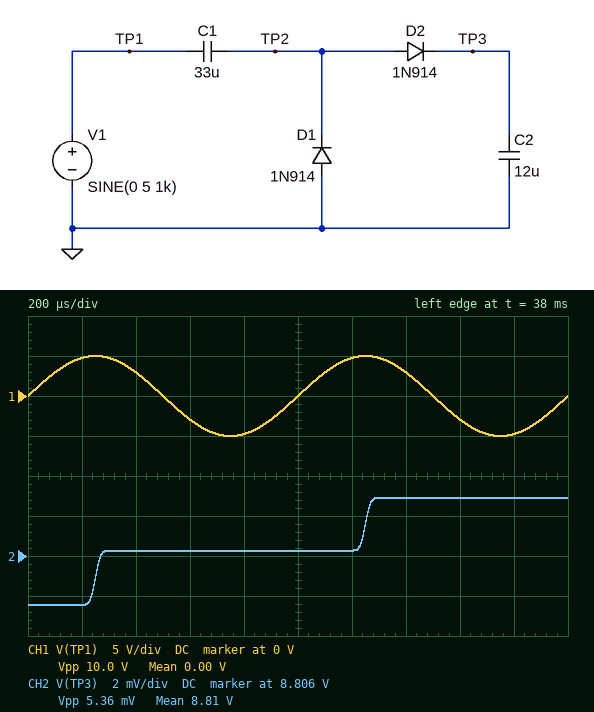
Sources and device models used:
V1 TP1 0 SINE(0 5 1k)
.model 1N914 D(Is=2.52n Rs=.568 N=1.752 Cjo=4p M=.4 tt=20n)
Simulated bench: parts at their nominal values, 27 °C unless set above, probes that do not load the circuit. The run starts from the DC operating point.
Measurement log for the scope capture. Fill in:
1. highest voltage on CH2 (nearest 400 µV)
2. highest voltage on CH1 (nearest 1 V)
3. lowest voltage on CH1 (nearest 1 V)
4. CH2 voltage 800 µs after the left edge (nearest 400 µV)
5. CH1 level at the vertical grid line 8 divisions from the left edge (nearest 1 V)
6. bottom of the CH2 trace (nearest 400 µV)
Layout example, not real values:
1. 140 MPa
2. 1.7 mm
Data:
1. 8.8088 V
2. 5 V
3. -5 V
4. 8.8064 V
5. -3 V
6. 8.8036 V
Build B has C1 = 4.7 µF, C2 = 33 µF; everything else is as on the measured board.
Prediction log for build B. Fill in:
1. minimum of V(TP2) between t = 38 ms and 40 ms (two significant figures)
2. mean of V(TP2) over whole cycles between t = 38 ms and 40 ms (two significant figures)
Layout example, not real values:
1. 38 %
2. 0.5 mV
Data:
1. -680 mV
2. 4.3 V
